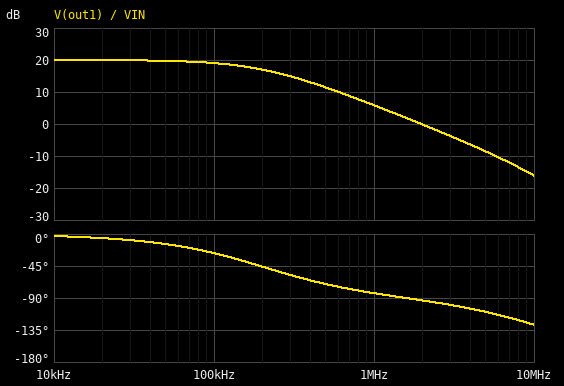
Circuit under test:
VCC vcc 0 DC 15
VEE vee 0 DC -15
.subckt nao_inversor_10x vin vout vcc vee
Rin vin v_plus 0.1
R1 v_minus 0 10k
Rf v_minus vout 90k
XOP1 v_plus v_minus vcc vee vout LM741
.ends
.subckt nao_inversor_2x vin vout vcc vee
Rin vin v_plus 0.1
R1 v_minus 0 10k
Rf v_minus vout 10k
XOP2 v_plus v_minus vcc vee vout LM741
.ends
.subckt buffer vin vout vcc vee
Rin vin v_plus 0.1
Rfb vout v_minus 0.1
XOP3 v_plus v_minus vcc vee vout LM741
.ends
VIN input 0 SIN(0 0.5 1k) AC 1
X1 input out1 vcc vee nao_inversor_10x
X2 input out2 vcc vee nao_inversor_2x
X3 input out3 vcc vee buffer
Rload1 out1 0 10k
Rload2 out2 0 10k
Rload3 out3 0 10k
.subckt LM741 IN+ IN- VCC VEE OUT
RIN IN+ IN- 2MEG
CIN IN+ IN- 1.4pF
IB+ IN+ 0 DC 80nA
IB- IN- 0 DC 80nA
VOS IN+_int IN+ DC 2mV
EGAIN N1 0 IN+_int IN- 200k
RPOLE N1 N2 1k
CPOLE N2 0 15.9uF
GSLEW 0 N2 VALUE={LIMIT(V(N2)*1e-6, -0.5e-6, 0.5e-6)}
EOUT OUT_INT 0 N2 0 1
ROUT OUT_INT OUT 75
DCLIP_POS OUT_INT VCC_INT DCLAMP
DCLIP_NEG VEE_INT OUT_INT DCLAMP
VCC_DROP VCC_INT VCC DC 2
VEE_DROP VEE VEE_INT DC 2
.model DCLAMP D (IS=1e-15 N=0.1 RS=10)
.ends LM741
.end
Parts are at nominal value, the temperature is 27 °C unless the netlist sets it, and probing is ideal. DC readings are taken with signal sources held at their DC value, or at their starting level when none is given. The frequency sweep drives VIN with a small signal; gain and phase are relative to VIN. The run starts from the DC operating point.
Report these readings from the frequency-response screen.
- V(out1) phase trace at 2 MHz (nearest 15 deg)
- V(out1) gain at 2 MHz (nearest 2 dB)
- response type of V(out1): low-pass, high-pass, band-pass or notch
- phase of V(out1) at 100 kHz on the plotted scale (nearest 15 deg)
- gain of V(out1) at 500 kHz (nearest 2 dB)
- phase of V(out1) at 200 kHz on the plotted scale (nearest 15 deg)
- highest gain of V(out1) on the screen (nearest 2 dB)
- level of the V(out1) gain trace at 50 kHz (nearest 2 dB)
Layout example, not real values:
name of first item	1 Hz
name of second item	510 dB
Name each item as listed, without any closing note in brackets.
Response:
V(out1) phase trace at 2 MHz	-90 deg
V(out1) gain at 2 MHz	0 dB
response type of V(out1): low-pass, high-pass, band-pass or notch	low-pass
phase of V(out1) at 100 kHz on the plotted scale	-30 deg
gain of V(out1) at 500 kHz	12 dB
phase of V(out1) at 200 kHz on the plotted scale	-45 deg
highest gain of V(out1) on the screen	20 dB
level of the V(out1) gain trace at 50 kHz	20 dB
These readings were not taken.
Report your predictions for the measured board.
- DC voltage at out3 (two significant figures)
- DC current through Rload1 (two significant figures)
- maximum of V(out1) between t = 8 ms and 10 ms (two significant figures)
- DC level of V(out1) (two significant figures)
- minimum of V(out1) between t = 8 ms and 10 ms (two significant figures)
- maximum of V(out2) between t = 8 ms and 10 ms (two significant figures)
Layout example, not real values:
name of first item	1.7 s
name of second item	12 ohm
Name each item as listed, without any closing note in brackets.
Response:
DC voltage at out3	2.0 mV
DC current through Rload1	2.7 µA
maximum of V(out1) between t = 8 ms and 10 ms	5.0 V
DC level of V(out1)	27 mV
minimum of V(out1) between t = 8 ms and 10 ms	-5.0 V
maximum of V(out2) between t = 8 ms and 10 ms	1.0 V
